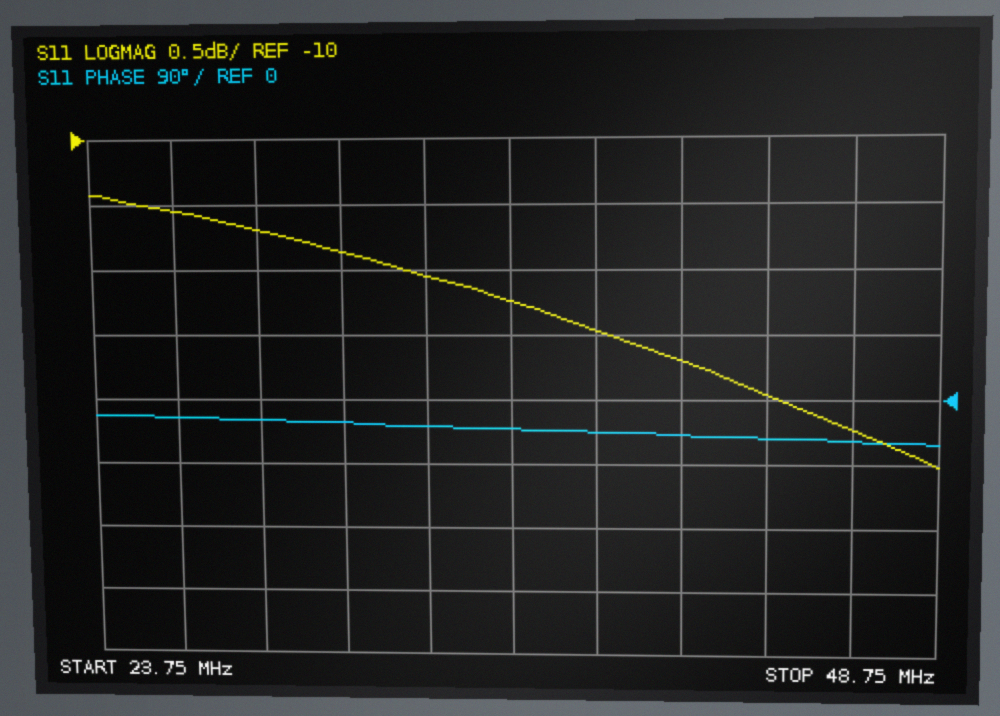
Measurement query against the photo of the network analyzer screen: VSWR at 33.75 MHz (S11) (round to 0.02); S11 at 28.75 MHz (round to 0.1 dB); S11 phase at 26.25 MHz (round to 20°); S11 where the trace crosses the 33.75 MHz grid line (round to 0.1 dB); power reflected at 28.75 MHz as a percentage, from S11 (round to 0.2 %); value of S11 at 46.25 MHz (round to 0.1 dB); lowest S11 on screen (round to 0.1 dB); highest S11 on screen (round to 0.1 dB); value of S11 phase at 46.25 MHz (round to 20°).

1.78
-10.7 dB
-20°
-11.0 dB
8.6 %
-12.2 dB
-12.5 dB
-10.4 dB
-60°
